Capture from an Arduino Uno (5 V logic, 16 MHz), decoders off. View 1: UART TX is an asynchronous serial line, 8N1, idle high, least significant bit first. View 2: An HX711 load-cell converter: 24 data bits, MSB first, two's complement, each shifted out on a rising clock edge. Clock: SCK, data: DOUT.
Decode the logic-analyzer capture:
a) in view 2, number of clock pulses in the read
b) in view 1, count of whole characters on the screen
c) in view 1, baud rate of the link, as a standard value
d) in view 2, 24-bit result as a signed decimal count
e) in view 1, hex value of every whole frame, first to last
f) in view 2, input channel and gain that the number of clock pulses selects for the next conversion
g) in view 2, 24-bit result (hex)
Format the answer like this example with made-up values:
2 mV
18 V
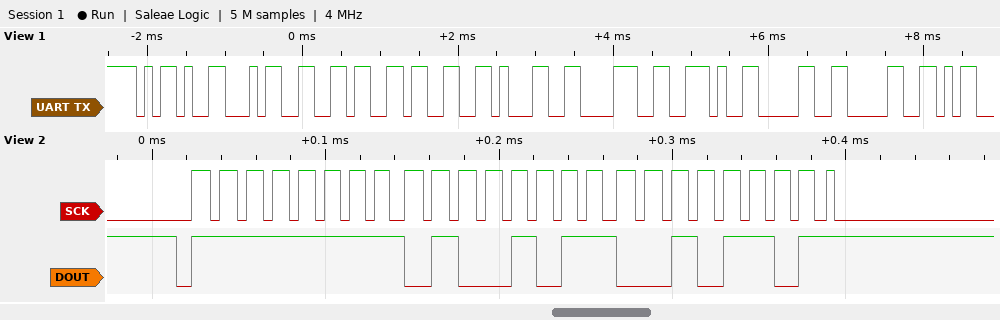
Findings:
25
9
9600 baud
-46291
2D 34 36 33 31 38 2E 30 30
channel A, gain 128
0xFF4B2D
